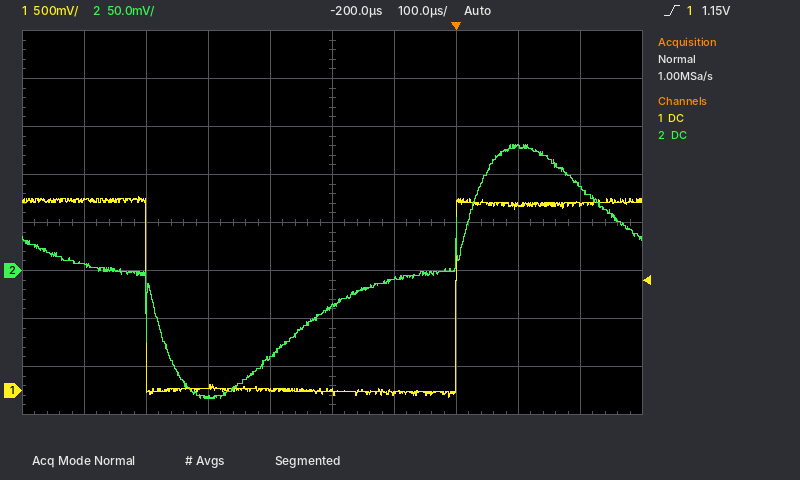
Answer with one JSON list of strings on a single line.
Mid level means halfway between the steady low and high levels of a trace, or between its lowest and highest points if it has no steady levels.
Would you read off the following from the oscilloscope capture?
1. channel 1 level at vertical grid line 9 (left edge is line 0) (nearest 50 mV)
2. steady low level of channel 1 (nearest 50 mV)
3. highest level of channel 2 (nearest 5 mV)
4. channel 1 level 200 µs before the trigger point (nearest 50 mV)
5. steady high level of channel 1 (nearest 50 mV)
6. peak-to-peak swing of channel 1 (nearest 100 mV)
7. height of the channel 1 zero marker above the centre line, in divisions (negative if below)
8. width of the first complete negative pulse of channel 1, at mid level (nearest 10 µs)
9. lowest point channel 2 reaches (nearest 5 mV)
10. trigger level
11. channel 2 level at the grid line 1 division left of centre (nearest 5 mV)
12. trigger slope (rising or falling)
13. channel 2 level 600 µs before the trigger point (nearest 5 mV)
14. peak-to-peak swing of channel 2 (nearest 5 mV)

["1.95 V", "0 mV", "130 mV", "0 mV", "1.95 V", "2.10 V", "-3.5 div", "500 µs", "-135 mV", "1.15 V", "-90 mV", "rising", "5 mV", "265 mV"]
